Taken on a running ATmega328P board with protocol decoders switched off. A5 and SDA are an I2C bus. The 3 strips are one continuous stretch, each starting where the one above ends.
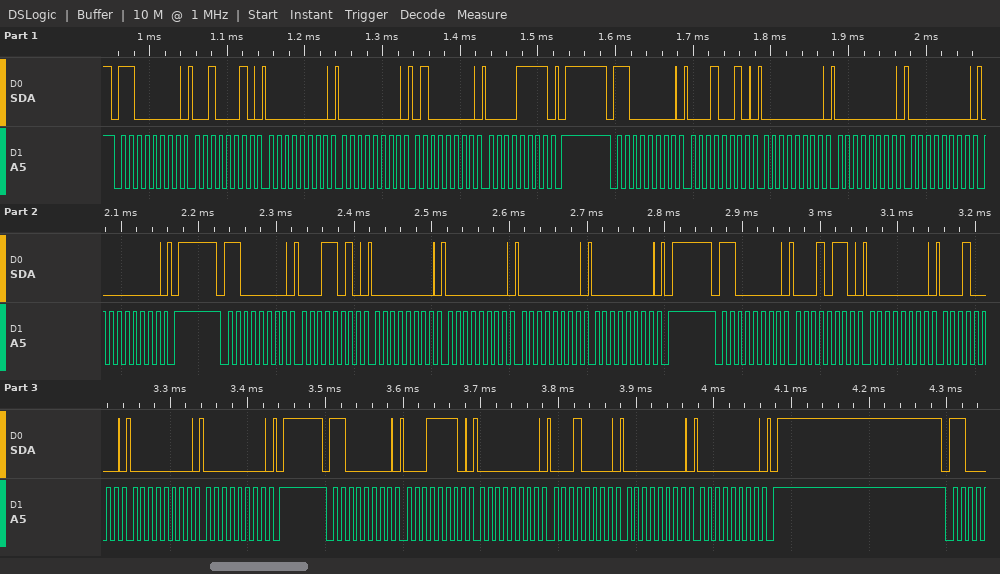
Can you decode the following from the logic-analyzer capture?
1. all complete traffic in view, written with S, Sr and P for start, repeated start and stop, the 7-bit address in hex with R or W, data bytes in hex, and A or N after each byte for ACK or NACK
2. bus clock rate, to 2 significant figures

S 60W A 22 A 00 A 00 A 40 A 0F A P S 60W A 12 A 00 A 00 A 00 A 00 A P S 60W A 1A A 00 A 00 A 00 A 00 A P S 60W A 16 A 00 A 10 A 00 A 00 A P S 60W A 1E A 00 A 10 A 00 A 00 A P
100 kHz
